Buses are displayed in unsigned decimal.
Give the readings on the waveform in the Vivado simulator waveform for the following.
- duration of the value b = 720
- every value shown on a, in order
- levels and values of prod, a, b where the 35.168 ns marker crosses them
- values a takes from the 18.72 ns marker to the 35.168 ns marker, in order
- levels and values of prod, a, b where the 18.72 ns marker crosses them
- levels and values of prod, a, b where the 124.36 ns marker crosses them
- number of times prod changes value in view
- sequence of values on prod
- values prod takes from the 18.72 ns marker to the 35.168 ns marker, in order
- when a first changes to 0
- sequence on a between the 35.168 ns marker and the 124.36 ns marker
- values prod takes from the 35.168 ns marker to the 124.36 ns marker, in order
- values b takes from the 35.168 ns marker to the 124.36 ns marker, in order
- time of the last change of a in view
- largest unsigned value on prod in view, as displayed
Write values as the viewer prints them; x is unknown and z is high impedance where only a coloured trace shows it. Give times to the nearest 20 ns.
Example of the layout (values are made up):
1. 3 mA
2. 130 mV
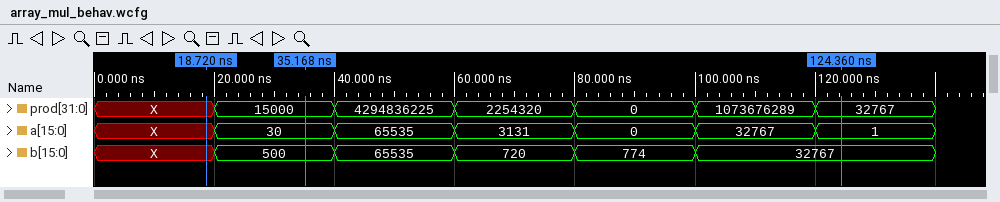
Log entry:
1. 20 ns
2. X, 30, 65535, 3131, 0, 32767, 1
3. prod=15000, a=30, b=500
4. X, 30
5. prod=X, a=X, b=X
6. prod=32767, a=1, b=32767
7. 6
8. X, 15000, 4294836225, 2254320, 0, 1073676289, 32767
9. X, 15000
10. 80 ns
11. 30, 65535, 3131, 0, 32767, 1
12. 15000, 4294836225, 2254320, 0, 1073676289, 32767
13. 500, 65535, 720, 774, 32767
14. 120 ns
15. 4294836225
